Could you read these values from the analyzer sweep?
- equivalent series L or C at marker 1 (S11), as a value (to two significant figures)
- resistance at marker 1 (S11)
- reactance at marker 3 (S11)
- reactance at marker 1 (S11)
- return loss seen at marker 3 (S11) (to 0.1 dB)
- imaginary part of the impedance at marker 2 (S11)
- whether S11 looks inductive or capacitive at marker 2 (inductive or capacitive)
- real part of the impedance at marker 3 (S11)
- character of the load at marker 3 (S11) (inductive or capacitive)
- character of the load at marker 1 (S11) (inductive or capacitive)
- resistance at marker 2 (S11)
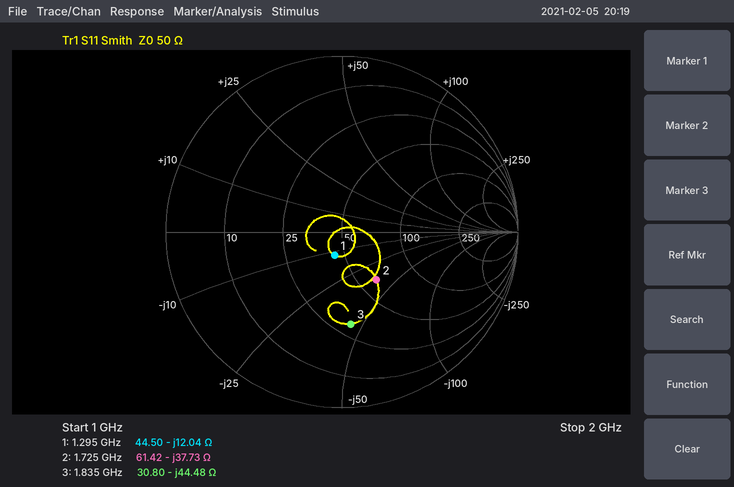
10 pF
44.50 Ω
-44.48 Ω
-12.04 Ω
5.6 dB
-37.73 Ω
capacitive
30.80 Ω
capacitive
capacitive
61.42 Ω
